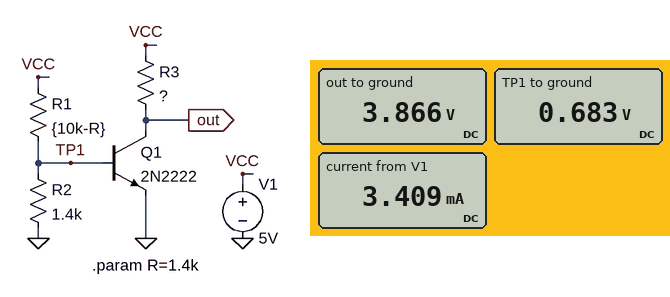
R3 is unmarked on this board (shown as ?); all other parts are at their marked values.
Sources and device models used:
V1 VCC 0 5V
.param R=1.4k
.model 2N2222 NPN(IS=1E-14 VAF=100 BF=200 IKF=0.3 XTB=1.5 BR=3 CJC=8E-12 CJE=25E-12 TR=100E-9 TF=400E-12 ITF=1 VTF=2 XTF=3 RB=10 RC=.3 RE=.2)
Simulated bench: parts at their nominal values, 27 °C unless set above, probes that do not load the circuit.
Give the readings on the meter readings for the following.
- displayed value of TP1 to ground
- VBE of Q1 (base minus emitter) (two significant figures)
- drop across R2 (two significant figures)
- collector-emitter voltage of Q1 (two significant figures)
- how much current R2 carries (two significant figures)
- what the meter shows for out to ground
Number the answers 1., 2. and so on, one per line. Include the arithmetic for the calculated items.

1. 0.683 V
2. 683 mV = 680 mV
3. 683 mV = 680 mV
4. 3.866 V = 3.9 V
5. (683 mV) / 1.4 kΩ = 490 µA
6. 3.866 V
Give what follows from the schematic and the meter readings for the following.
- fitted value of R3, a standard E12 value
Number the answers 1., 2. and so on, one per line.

1. 390 Ω
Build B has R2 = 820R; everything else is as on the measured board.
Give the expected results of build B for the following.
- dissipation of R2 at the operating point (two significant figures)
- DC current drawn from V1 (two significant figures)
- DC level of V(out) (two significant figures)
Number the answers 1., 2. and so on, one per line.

1. 230 µW
2. 530 µA
3. 5.0 V
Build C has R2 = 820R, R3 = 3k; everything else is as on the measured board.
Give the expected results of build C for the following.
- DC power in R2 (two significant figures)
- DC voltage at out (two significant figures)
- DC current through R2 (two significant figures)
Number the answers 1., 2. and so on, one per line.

1. 230 µW
2. 5.0 V
3. 530 µA
